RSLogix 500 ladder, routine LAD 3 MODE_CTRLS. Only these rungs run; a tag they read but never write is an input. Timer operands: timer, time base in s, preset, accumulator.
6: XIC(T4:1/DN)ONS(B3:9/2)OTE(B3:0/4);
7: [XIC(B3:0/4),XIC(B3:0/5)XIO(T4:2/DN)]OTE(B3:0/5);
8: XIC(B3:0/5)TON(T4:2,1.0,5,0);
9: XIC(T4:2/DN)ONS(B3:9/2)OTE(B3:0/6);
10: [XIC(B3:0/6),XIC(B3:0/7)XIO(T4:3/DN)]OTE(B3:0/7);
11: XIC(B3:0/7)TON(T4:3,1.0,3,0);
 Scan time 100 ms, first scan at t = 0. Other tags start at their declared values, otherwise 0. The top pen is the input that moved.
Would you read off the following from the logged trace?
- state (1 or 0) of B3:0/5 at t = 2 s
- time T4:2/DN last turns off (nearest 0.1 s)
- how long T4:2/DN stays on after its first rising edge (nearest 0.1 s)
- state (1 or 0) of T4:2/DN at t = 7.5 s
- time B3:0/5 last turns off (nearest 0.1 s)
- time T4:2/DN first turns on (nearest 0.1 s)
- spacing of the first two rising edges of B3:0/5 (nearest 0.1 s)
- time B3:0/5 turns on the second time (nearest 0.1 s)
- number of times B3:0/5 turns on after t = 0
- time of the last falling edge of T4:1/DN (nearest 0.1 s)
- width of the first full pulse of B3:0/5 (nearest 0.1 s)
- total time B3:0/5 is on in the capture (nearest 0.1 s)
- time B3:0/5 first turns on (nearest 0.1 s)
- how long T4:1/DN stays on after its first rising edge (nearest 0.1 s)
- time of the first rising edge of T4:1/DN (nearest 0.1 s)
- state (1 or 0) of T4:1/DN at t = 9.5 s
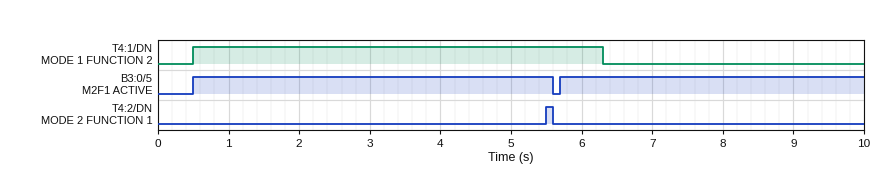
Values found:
1
5.6 s
0.1 s
0
5.6 s
5.5 s
5.2 s
5.7 s
2
6.3 s
5.1 s
9.4 s
0.5 s
5.8 s
0.5 s
0
